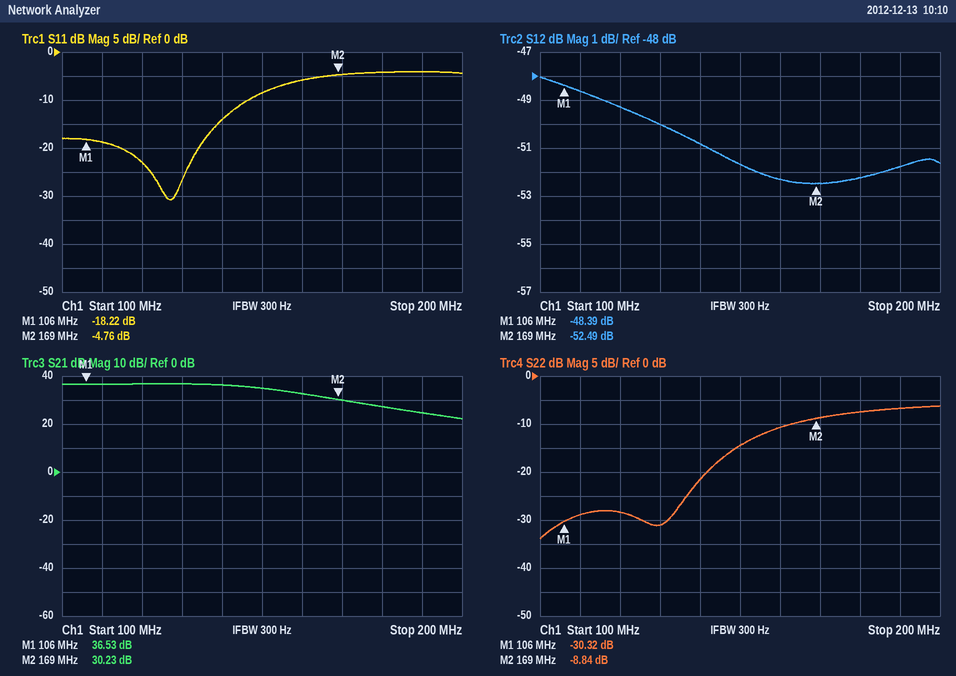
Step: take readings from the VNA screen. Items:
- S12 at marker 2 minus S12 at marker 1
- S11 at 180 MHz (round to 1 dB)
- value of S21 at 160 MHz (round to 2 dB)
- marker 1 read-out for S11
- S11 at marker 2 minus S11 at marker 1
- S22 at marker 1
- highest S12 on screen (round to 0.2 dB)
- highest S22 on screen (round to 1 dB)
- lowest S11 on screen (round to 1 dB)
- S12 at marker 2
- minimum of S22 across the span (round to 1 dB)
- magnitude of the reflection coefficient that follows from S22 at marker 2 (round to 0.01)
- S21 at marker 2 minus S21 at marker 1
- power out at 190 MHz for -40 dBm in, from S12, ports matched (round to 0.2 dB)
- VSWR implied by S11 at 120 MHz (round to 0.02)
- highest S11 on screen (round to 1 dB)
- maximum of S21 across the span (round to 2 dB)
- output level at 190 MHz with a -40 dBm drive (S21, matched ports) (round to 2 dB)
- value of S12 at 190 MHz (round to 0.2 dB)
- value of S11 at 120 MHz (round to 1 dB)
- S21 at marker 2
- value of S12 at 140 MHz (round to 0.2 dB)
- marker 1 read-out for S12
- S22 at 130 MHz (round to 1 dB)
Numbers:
-4.10 dB
-4 dB
32 dB
-18.22 dB
13.46 dB
-30.32 dB
-48.0 dB
-6 dB
-31 dB
-52.49 dB
-34 dB
0.36
-6.30 dB
-91.8 dBm
1.16
-4 dB
36 dB
-16 dBm
-51.8 dB
-23 dB
30.23 dB
-50.8 dB
-48.39 dB
-31 dB
